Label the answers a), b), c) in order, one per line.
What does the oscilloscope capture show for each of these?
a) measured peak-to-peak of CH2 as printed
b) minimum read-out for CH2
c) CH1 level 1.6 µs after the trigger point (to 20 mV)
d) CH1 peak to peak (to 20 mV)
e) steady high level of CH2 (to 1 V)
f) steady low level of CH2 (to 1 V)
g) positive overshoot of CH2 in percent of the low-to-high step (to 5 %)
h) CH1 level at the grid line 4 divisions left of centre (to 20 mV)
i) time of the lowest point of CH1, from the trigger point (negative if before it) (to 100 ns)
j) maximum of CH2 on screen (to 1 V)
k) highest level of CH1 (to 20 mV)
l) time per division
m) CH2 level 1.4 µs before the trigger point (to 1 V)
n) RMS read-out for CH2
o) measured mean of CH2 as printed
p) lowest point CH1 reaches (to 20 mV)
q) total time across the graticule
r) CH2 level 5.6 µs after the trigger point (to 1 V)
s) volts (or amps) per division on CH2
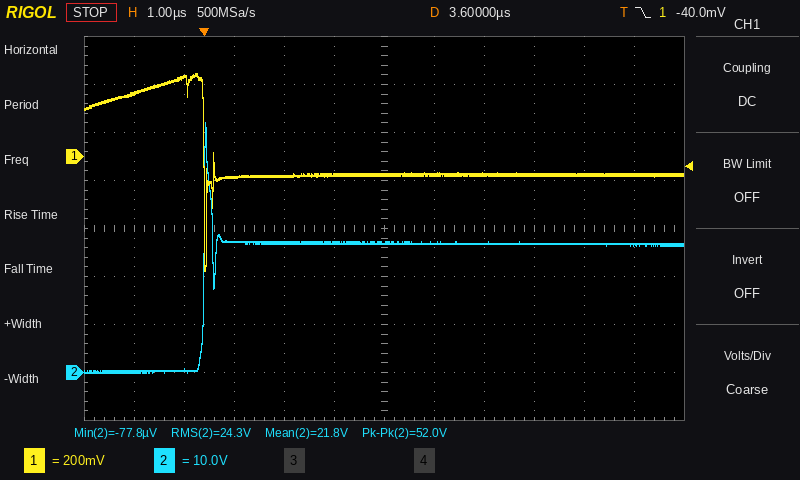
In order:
a) 52.0 V
b) -77.8 µV
c) -80 mV
d) 820 mV
e) 27 V
f) 0 V
g) 95 %
h) 320 mV
i) 0.0 µs
j) 52 V
k) 340 mV
l) 1 µs
m) 0 V
n) 24.3 V
o) 21.8 V
p) -480 mV
q) 12 µs
r) 27 V
s) 10 V
